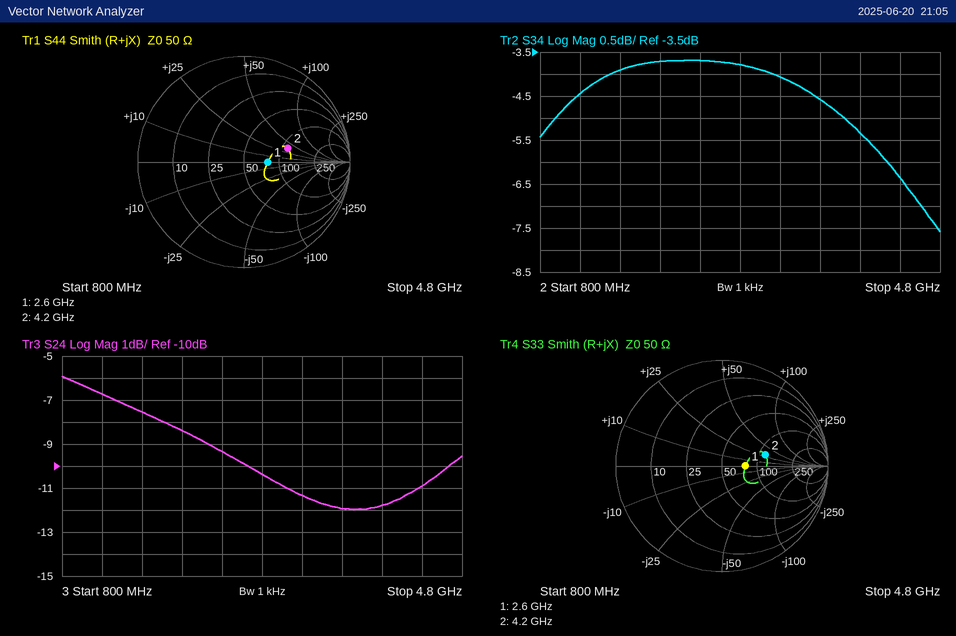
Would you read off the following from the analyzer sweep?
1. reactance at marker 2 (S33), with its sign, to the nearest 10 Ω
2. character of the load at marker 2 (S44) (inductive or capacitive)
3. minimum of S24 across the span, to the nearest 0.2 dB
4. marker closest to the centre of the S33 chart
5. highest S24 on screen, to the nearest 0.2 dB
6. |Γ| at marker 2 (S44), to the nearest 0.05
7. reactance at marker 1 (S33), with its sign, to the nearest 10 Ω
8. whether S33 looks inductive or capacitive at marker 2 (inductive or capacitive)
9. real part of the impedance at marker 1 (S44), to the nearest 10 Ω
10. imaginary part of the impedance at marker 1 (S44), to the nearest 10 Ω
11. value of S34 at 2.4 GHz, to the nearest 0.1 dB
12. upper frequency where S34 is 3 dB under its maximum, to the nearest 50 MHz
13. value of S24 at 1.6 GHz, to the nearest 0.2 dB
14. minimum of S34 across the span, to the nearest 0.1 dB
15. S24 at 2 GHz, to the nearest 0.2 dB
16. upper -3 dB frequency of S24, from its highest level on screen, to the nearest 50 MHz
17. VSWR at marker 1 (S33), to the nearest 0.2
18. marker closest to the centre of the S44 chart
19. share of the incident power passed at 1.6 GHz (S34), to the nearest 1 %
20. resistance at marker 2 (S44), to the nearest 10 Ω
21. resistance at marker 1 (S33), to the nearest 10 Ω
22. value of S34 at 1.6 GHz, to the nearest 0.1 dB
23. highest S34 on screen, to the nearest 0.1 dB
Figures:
+30 Ω
inductive
-12.0 dB
marker 1
-6.0 dB
0.45
0 Ω
inductive
80 Ω
0 Ω
-3.7 dB
4.50 GHz
-7.6 dB
-7.6 dB
-8.4 dB
2.25 GHz
1.6
marker 1
41 %
110 Ω
80 Ω
-3.9 dB
-3.7 dB
